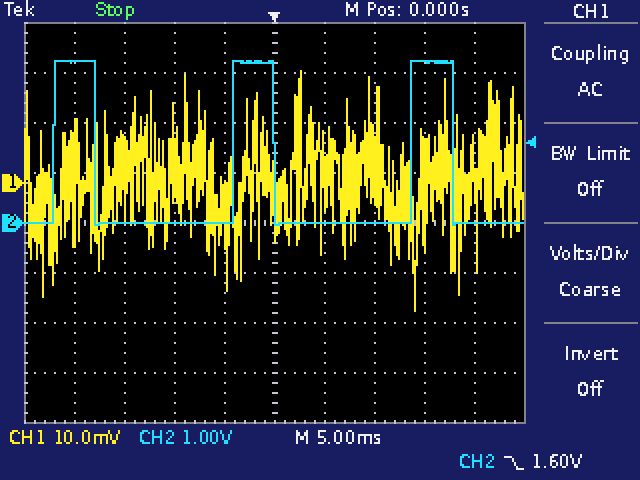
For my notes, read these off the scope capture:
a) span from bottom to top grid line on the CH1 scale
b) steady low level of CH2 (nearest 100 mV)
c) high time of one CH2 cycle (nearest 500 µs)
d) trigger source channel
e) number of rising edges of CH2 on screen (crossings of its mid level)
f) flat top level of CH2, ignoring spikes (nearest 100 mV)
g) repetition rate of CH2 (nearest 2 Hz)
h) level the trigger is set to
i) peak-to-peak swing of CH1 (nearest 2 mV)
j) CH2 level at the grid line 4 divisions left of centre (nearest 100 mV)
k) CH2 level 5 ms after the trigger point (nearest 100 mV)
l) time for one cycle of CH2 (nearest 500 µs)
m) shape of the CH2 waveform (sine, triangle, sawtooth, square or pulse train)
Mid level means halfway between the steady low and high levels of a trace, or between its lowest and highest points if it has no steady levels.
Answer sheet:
80 mV
0.0 V
4.0 ms
CH2
3
3.2 V
56 Hz
1.60 V
48 mV
3.2 V
0.0 V
18.0 ms
pulse train
